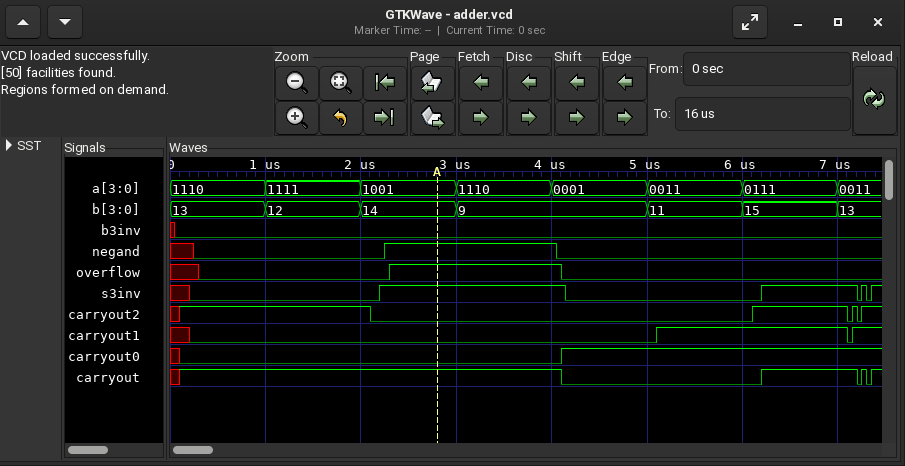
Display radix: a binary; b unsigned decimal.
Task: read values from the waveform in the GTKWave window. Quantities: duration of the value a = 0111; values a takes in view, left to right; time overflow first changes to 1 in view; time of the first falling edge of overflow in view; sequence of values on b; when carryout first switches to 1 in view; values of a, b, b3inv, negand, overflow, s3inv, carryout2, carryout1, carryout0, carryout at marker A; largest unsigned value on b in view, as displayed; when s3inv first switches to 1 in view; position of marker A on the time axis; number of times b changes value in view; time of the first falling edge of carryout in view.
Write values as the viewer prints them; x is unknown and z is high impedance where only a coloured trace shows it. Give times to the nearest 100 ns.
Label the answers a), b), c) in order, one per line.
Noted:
a) 1000 ns
b) 1110, 1111, 1001, 1110, 0001, 0011, 0111, 0011
c) 2300 ns
d) 4100 ns
e) 13, 12, 14, 9, 11, 15, 13
f) 100 ns
g) a=1001, b=14, b3inv=0, negand=1, overflow=1, s3inv=1, carryout2=0, carryout1=0, carryout0=0, carryout=1
h) 15
i) 2200 ns
j) 2800 ns
k) 6
l) 4100 ns
